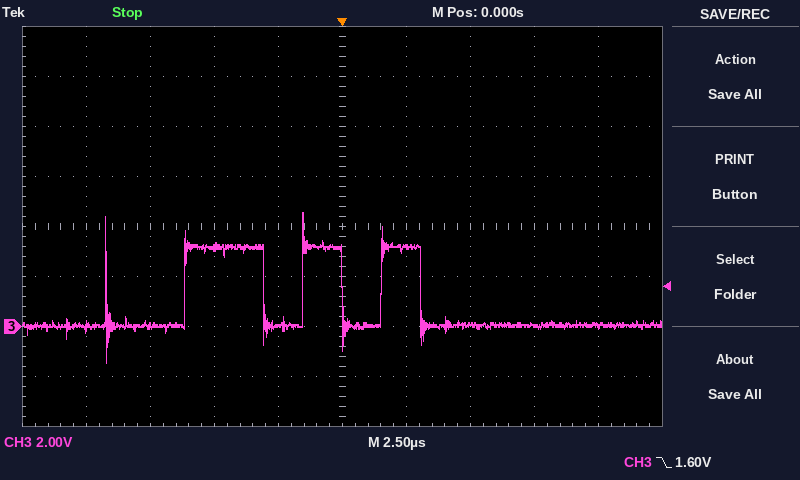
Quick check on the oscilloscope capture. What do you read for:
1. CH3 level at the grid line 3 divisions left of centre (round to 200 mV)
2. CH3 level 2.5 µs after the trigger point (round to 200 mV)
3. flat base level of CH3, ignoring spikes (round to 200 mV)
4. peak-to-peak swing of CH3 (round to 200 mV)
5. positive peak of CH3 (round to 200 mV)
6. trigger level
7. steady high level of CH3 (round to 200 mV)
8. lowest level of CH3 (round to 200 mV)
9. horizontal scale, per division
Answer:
0.0 V
3.2 V
0.0 V
6.0 V
4.6 V
1.60 V
3.2 V
-1.4 V
2.5 µs
